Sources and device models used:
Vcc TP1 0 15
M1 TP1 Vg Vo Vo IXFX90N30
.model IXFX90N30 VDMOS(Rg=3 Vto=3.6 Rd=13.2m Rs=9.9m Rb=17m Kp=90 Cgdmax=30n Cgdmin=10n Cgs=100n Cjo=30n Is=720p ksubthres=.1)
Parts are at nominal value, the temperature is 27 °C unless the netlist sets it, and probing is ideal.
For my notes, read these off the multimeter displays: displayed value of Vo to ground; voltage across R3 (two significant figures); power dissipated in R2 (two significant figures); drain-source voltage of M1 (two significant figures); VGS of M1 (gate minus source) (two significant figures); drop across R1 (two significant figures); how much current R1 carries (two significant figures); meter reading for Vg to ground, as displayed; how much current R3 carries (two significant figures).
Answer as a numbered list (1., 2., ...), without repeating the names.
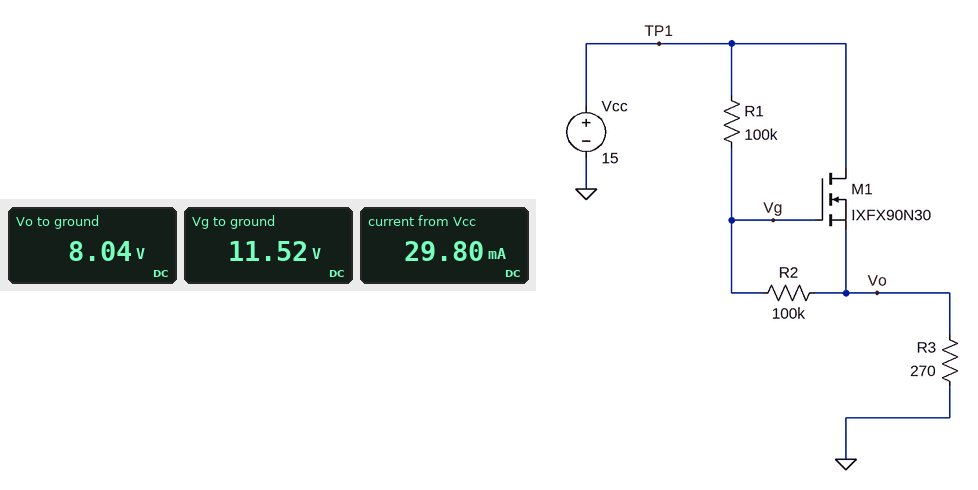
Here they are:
1. 8.04 V
2. 8.0 V
3. 120 µW
4. 7.0 V
5. 3.5 V
6. 3.5 V
7. 35 µA
8. 11.52 V
9. 30 mA
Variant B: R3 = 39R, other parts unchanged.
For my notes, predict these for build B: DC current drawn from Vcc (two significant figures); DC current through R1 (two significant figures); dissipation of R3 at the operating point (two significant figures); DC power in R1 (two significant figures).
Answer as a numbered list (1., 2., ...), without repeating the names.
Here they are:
1. 200 mA
2. 36 µA
3. 1.6 W
4. 130 µW
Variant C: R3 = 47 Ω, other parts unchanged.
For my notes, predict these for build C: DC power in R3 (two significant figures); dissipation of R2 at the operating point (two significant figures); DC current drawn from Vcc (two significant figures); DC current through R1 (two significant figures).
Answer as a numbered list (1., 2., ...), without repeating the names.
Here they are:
1. 1.3 W
2. 130 µW
3. 170 mA
4. 36 µA
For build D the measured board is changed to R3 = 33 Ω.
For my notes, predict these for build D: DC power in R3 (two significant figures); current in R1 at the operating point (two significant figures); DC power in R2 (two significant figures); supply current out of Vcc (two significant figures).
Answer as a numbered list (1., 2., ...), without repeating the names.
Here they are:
1. 1.8 W
2. 36 µA
3. 130 µW
4. 240 mA
